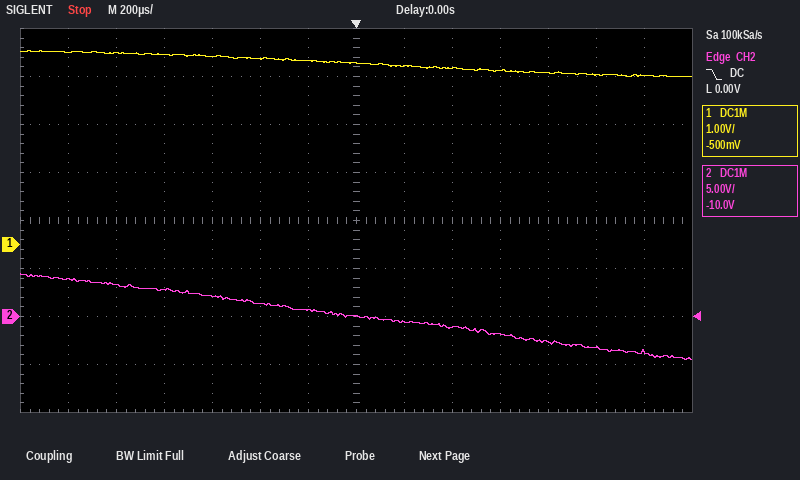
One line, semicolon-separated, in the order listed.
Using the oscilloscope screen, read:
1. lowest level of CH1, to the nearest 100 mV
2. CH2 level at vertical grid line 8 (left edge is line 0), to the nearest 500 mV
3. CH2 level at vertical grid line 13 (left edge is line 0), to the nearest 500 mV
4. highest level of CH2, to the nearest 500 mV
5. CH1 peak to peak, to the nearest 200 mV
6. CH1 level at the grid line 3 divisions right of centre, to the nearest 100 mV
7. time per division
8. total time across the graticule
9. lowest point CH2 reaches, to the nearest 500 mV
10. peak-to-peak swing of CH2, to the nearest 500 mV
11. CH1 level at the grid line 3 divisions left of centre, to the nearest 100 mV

3.5 V; -500 mV; -3.5 V; 4.5 V; 600 mV; 3.6 V; 200 µs; 2.8 ms; -4.5 V; 9.0 V; 3.9 V
